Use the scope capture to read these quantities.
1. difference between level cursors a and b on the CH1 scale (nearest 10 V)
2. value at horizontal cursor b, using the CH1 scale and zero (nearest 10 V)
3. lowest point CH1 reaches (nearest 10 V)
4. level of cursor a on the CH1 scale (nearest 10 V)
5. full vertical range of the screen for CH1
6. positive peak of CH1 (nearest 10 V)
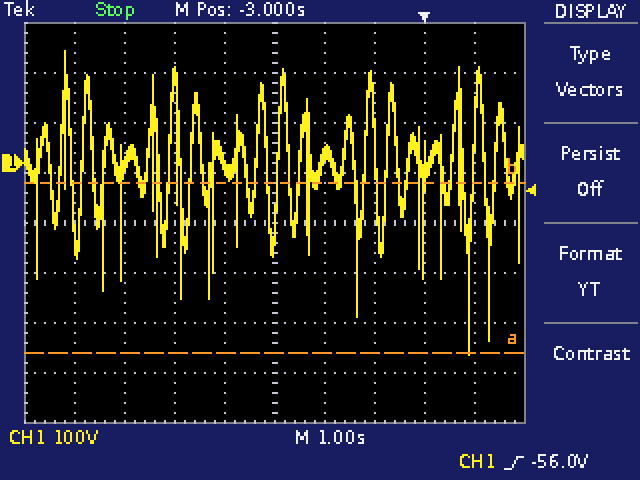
340 V
-40 V
-380 V
-380 V
800 V
220 V
